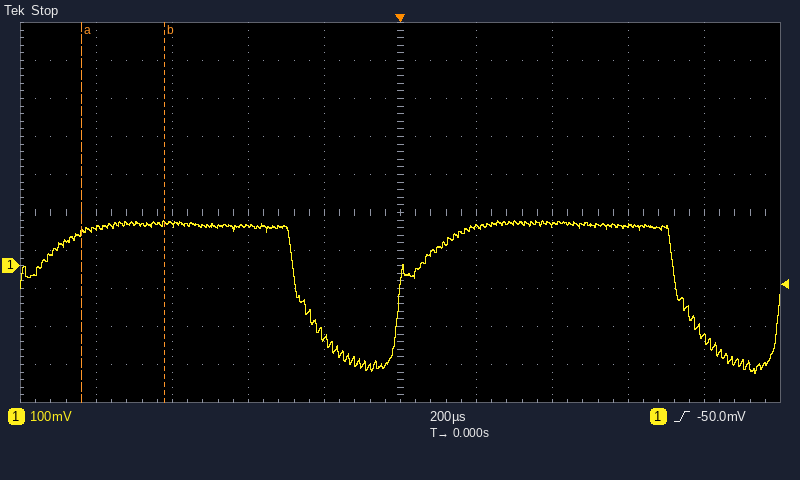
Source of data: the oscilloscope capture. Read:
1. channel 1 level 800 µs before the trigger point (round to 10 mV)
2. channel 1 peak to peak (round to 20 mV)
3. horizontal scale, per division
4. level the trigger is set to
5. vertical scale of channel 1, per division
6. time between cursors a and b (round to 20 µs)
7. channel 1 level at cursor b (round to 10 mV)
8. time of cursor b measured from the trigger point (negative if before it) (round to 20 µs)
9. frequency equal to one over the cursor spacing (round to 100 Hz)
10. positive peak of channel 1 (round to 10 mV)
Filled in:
100 mV
400 mV
200 µs
-50.0 mV
100 mV
220 µs
110 mV
-620 µs
4.5 kHz
120 mV
